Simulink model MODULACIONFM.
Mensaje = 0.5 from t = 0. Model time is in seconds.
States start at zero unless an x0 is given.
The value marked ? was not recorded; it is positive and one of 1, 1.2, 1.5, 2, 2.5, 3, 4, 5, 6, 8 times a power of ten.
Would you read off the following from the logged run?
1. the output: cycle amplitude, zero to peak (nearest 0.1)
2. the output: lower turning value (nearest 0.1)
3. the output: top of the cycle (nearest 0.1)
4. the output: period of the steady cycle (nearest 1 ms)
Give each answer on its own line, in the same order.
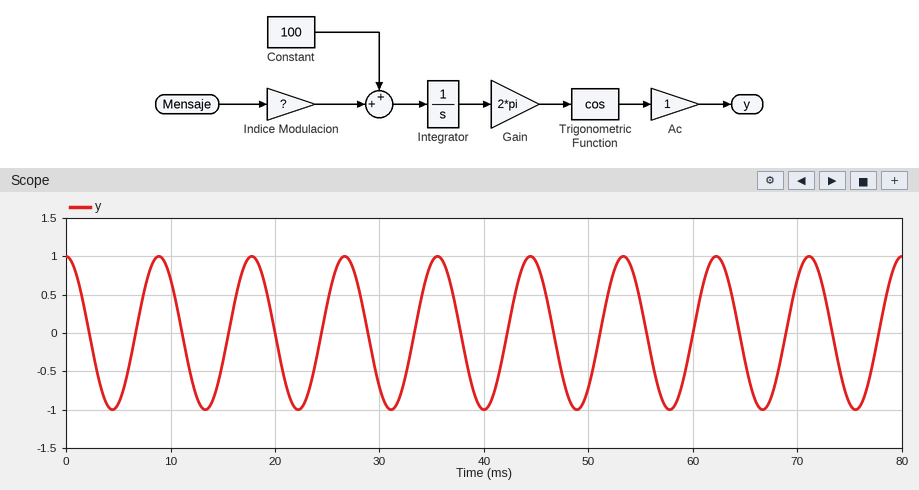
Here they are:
1.0
-1.0
1.0
9 ms
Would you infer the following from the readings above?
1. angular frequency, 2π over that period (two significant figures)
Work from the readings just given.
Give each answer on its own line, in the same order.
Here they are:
0.70 rad/ms
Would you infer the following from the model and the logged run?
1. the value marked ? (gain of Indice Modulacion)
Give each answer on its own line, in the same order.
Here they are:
25
